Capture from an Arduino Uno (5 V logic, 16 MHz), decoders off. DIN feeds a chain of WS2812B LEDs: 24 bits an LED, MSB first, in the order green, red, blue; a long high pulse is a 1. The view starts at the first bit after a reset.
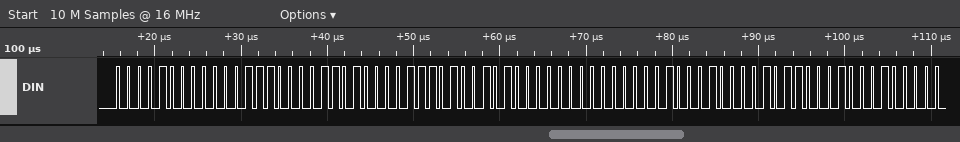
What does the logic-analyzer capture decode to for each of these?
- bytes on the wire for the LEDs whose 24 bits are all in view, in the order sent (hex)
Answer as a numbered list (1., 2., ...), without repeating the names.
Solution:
1. 08 0E 1A 1D 28 00 11 0B 11
